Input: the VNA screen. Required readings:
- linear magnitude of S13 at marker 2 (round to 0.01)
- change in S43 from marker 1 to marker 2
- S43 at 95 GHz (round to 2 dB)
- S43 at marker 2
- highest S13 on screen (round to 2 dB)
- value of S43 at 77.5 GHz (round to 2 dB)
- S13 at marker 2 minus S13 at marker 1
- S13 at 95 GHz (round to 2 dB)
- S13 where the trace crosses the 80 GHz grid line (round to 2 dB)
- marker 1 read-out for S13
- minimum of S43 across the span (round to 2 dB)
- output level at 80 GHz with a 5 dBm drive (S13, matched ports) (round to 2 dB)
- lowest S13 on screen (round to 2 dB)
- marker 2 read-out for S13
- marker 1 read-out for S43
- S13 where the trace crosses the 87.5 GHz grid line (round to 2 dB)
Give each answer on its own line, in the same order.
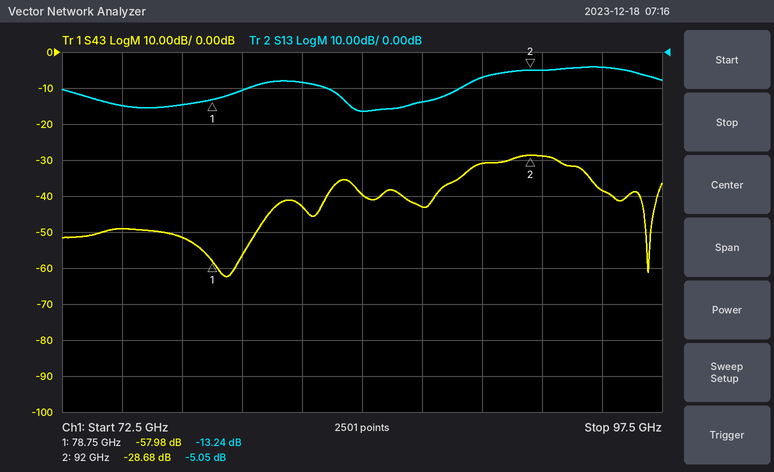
0.56
29.30 dB
-38 dB
-28.68 dB
-4 dB
-52 dB
8.19 dB
-4 dB
-10 dB
-13.24 dB
-62 dB
-6 dBm
-16 dB
-5.05 dB
-57.98 dB
-14 dB
